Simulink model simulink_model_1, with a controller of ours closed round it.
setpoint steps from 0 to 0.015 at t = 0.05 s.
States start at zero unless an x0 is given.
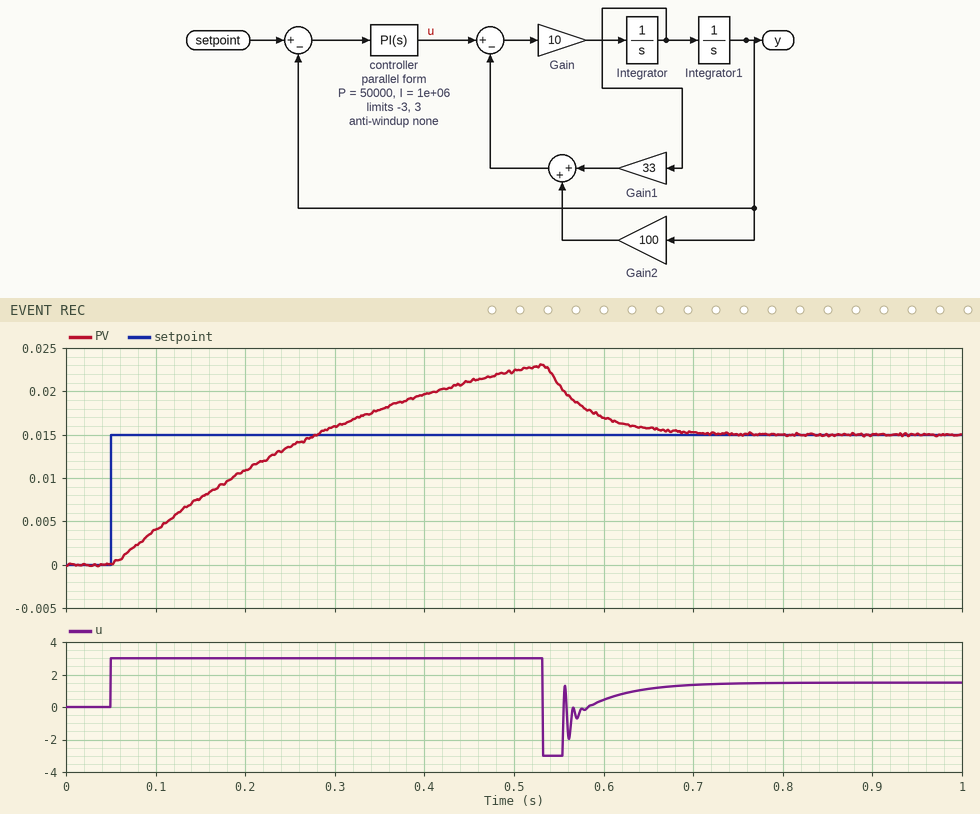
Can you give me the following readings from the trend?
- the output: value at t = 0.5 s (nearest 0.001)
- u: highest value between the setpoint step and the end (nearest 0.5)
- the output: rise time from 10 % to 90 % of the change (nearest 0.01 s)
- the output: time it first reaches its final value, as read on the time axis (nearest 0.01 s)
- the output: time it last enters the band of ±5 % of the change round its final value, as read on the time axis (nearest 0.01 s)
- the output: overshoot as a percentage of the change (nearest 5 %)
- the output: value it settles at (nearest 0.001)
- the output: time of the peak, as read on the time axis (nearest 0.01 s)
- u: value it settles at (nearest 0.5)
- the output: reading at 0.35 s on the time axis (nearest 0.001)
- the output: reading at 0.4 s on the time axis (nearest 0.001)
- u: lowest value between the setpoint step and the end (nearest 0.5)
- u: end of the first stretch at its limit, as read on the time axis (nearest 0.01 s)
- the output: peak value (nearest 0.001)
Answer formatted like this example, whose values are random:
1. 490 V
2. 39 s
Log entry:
1. 0.022
2. 3.0
3. 0.18 s
4. 0.28 s
5. 0.65 s
6. 55 %
7. 0.015
8. 0.53 s
9. 1.5
10. 0.018
11. 0.020
12. -3.0
13. 0.53 s
14. 0.023
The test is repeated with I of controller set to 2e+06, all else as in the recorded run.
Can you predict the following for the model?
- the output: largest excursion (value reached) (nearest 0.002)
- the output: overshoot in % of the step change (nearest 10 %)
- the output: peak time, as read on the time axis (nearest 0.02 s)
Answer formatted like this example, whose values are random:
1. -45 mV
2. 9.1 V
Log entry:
1. 0.024
2. 60 %
3. 0.56 s
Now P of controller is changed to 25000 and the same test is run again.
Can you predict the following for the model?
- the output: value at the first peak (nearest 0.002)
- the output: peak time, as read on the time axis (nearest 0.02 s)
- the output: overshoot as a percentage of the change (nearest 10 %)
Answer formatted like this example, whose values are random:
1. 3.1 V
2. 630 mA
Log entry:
1. 0.024
2. 0.56 s
3. 60 %
